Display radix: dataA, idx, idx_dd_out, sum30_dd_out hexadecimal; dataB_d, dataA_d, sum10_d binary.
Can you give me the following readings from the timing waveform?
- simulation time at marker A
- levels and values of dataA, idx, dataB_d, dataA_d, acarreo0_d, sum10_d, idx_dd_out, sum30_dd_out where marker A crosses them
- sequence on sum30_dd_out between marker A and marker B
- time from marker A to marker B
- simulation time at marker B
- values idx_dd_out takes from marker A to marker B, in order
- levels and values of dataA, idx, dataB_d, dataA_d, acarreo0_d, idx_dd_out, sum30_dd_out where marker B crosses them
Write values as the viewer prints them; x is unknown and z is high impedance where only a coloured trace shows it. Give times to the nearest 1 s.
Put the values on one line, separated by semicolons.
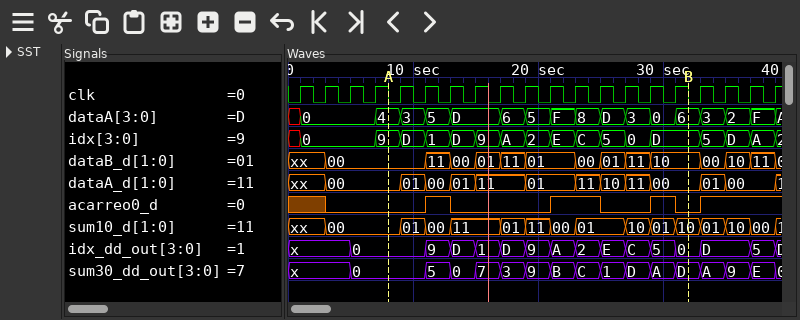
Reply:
8 s; dataA=4, idx=9, dataB_d=00, dataA_d=00, acarreo0_d=0, sum10_d=00, idx_dd_out=0, sum30_dd_out=0; 0, 5, 0, 7, 3, 9, B, C, 1, D, A, D; 24 s; 32 s; 0, 9, D, 1, D, 9, A, 2, E, C, 5, 0; dataA=6, idx=D, dataB_d=10, dataA_d=00, acarreo0_d=0, idx_dd_out=0, sum30_dd_out=D
